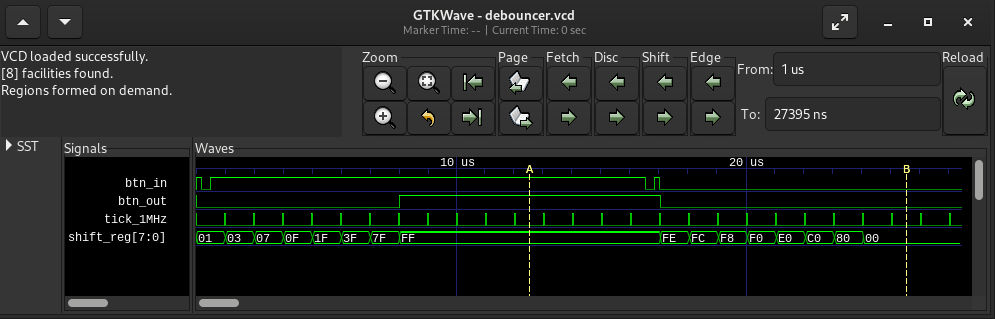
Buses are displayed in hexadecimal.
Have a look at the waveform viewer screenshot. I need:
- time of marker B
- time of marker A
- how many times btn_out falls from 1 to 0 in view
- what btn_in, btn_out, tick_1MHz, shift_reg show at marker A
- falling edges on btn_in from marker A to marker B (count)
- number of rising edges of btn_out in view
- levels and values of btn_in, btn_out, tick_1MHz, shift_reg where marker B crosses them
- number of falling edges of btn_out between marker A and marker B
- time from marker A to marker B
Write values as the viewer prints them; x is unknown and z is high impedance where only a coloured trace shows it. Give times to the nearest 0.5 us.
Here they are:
25.5 us
12.5 us
1
btn_in=1, btn_out=1, tick_1MHz=0, shift_reg=FF
2
1
btn_in=0, btn_out=0, tick_1MHz=0, shift_reg=00
1
13 us
